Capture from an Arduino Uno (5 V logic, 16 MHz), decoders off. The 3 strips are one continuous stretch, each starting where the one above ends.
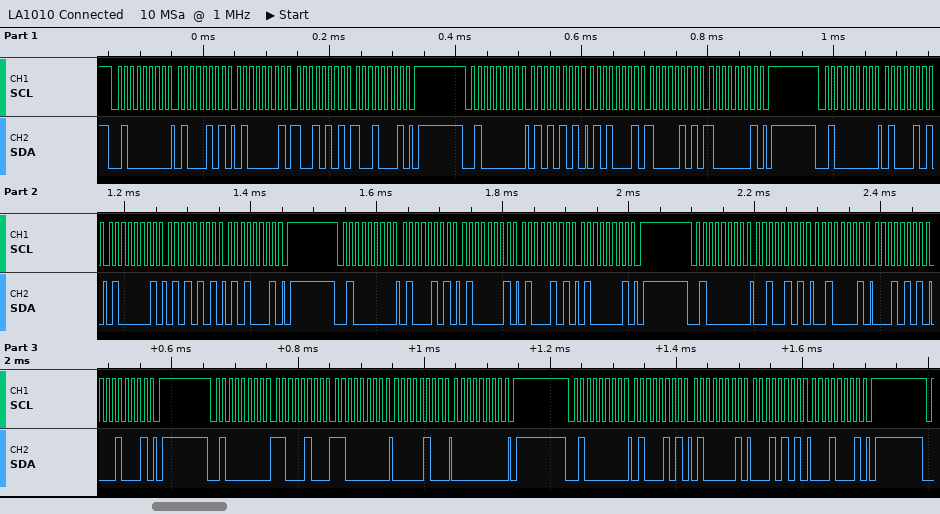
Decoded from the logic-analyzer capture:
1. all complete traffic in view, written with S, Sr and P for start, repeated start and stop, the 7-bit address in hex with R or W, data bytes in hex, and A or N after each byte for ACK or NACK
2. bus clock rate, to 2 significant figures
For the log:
S 20W A 45 A 41 A 95 A 91 A P S 20W A 55 A 51 A 85 A 81 A P S 20W A 45 A 41 A 55 A 51 A P S 20W A 45 A 41 A 45 A 41 A P S 20W A 25 A 21 A 15 A 11 A P S 20W A C4 A C0 A 04 A 00 A P S 20W A 45 A 41 A 15 A 11 A P
100 kHz
